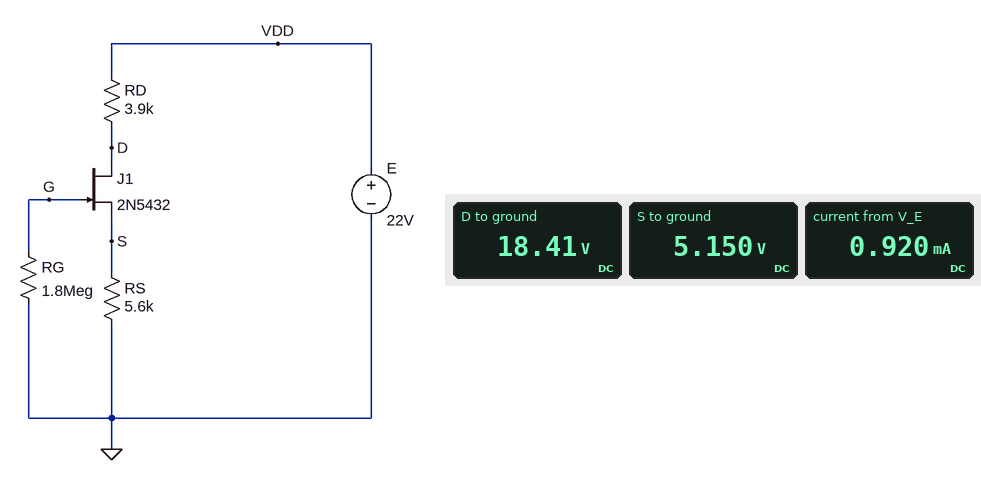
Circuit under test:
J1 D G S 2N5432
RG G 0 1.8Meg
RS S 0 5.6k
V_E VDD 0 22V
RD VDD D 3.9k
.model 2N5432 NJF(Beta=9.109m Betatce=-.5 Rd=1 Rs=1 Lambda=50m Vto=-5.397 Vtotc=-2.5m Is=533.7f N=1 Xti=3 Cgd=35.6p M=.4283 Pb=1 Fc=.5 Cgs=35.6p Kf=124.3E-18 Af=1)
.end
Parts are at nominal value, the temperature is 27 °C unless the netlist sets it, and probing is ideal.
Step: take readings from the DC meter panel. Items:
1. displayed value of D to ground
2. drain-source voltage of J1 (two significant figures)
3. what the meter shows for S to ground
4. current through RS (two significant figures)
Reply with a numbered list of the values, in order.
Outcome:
1. 18.41 V
2. 13 V
3. 5.150 V
4. 920 µA
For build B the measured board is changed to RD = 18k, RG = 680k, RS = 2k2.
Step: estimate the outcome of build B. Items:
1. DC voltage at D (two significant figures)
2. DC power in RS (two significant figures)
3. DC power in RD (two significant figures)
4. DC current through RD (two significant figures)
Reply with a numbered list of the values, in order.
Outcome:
1. 2.4 V
2. 2.6 mW
3. 21 mW
4. 1.1 mA
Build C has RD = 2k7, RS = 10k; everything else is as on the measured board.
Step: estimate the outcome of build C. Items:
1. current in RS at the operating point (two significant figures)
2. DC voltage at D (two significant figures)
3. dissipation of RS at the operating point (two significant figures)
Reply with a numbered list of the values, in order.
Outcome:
1. 520 µA
2. 21 V
3. 2.7 mW
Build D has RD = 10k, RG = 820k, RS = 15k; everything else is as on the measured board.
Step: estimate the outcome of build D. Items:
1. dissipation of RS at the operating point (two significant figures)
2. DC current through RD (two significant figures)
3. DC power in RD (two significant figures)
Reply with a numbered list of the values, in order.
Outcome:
1. 1.8 mW
2. 350 µA
3. 1.2 mW
